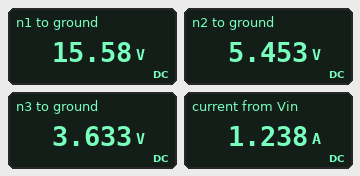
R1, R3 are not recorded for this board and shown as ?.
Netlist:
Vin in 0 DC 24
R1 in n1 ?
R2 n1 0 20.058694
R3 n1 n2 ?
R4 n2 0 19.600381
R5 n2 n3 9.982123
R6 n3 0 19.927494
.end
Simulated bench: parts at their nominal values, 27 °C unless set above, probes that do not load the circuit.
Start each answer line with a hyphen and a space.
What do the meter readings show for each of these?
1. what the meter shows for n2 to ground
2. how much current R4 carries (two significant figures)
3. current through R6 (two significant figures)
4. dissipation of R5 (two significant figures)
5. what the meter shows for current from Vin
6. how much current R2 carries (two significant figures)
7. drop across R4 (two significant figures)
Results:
- 5.453 V
- 280 mA
- 180 mA
- 330 mW
- 1.238 A
- 780 mA
- 5.5 V
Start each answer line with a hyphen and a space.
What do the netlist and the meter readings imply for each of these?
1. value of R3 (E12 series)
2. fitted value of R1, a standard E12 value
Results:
- 22 Ω
- 6.8 Ω
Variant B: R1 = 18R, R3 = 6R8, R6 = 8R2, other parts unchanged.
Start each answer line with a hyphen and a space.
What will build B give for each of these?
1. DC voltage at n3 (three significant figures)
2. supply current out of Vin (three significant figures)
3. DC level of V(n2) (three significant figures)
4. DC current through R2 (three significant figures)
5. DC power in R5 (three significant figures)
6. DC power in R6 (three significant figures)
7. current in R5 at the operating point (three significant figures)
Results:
- 2.09 V
- 890 mA
- 4.64 V
- 398 mA
- 650 mW
- 534 mW
- 255 mA
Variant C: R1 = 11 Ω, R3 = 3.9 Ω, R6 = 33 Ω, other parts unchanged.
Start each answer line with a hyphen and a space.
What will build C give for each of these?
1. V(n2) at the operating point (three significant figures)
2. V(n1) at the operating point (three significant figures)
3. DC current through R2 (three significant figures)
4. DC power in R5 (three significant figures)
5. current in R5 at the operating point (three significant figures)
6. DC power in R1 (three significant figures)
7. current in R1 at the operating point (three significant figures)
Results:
- 8.53 V
- 11.0 V
- 548 mA
- 393 mW
- 198 mA
- 15.4 W
- 1.18 A
